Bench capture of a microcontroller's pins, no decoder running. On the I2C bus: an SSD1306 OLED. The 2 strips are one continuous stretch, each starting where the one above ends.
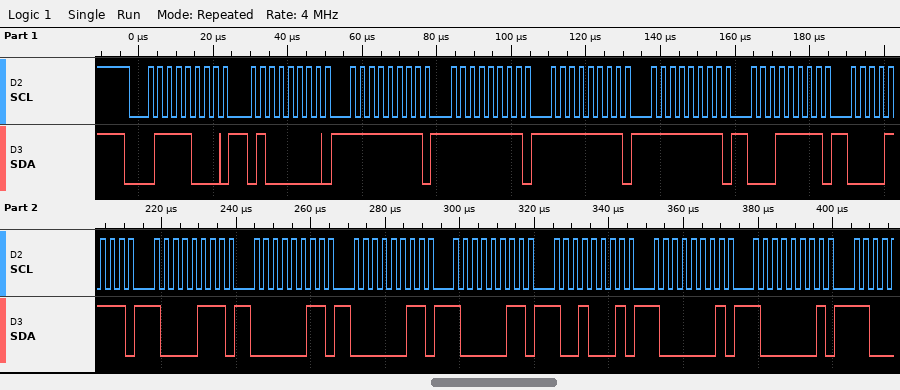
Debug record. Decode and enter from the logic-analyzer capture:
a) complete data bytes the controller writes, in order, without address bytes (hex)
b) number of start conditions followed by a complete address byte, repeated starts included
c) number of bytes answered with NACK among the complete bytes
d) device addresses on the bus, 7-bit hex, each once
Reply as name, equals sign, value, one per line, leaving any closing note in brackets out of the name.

complete data bytes the controller writes, in order, without address bytes = 40 FF FF FF FF 1F 0F 87 03 03 83 91 81 81
number of start conditions followed by a complete address byte, repeated starts included = 1
number of bytes answered with NACK among the complete bytes = 0
device addresses on the bus, 7-bit hex, each once = 0x3C
